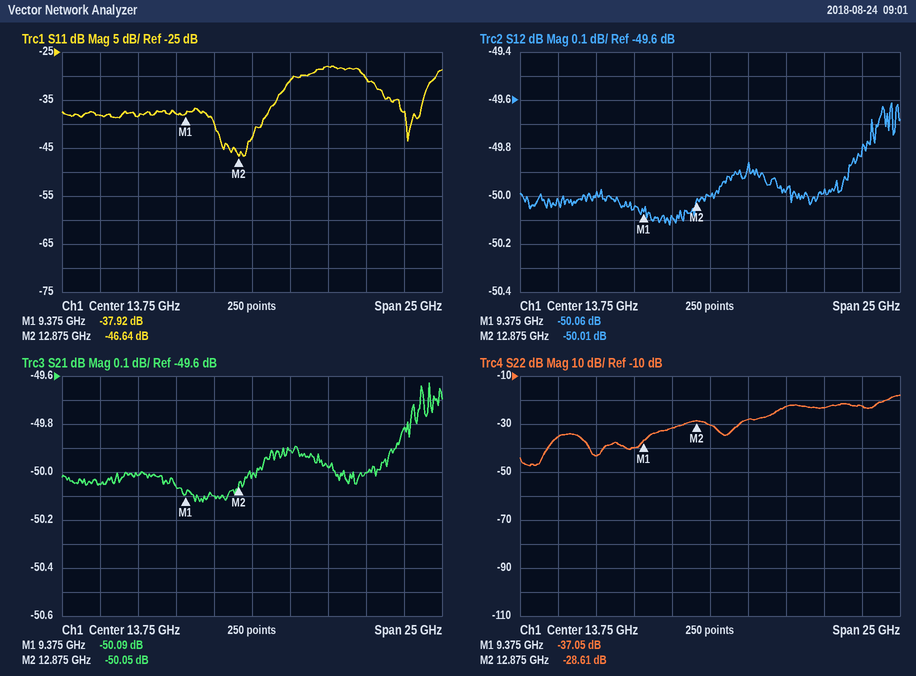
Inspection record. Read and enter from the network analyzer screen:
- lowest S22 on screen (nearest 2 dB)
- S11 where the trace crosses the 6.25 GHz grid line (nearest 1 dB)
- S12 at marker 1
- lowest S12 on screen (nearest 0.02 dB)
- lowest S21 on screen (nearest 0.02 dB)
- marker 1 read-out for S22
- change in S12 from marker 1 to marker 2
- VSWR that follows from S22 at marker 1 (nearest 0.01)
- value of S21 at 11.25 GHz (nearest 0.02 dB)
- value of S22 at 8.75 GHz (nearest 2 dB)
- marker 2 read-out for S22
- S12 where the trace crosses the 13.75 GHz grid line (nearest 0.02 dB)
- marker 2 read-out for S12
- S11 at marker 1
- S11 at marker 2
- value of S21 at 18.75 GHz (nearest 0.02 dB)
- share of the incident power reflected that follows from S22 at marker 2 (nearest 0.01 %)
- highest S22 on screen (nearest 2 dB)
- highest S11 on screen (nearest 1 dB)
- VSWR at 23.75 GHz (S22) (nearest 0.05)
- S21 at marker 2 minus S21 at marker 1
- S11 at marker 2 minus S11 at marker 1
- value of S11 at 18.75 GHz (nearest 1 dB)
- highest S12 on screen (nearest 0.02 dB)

-48 dB
-38 dB
-50.06 dB
-50.12 dB
-50.12 dB
-37.05 dB
0.05 dB
1.03
-50.10 dB
-40 dB
-28.61 dB
-50.00 dB
-50.01 dB
-37.92 dB
-46.64 dB
-49.98 dB
0.14 %
-18 dB
-28 dB
1.15
0.04 dB
-8.72 dB
-28 dB
-49.62 dB
